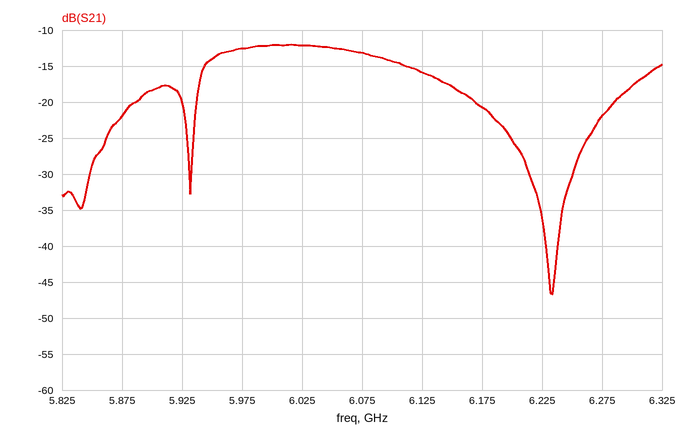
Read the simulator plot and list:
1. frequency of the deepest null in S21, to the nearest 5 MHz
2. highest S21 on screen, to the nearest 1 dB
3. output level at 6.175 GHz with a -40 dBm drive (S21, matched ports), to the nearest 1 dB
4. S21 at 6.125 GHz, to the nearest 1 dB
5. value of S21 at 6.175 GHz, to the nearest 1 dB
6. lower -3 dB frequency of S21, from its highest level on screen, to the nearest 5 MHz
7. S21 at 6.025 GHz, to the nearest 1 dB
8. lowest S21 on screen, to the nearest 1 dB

6.235 GHz
-12 dB
-61 dBm
-16 dB
-21 dB
5.945 GHz
-12 dB
-47 dB
